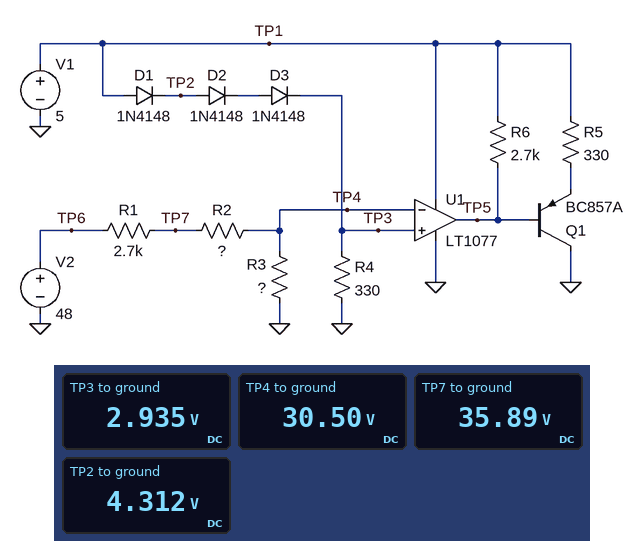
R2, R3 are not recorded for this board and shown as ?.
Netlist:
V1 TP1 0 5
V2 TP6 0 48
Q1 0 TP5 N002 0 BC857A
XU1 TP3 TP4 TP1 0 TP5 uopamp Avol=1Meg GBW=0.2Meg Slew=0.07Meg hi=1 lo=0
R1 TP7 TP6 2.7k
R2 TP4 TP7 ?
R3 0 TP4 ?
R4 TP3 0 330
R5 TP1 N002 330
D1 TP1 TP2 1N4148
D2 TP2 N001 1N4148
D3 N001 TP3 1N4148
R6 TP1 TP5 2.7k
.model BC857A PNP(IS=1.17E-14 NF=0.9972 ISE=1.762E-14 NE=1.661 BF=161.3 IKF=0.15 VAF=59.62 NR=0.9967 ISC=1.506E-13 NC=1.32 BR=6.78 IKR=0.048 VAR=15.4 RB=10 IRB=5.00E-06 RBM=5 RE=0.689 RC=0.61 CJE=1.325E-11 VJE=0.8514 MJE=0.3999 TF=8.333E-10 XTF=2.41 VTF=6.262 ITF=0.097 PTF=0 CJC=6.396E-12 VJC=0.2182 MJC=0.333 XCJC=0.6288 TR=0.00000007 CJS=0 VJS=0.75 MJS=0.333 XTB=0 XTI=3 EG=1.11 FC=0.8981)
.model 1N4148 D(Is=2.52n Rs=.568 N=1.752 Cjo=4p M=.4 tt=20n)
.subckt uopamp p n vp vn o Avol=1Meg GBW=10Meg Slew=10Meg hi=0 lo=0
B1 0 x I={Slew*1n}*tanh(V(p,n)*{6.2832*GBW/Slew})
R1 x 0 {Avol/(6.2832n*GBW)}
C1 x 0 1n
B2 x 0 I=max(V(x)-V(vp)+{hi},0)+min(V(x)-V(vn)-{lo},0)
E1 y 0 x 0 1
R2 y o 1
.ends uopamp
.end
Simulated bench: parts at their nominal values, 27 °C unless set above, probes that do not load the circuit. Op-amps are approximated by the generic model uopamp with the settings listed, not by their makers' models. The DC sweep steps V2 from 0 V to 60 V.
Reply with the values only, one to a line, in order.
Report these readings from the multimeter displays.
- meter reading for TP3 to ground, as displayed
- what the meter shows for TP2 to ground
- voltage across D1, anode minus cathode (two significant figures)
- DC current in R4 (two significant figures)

2.935 V
4.312 V
690 mV
8.9 mA
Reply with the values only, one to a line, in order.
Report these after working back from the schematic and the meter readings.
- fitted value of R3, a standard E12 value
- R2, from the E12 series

6.8 kΩ
1.2 kΩ
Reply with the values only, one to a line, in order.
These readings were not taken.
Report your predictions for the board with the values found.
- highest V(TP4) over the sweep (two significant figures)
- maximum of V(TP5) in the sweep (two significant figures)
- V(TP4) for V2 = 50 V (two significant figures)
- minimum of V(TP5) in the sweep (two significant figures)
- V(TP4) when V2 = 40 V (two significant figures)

38 V
4.0 V
32 V
1.9 mV
25 V
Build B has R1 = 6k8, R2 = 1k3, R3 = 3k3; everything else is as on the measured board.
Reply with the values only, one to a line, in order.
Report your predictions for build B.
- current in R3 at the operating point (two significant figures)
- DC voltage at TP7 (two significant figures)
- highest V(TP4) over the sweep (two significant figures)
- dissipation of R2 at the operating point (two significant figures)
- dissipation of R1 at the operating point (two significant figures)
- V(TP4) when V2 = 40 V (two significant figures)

4.2 mA
19 V
17 V
23 mW
120 mW
12 V
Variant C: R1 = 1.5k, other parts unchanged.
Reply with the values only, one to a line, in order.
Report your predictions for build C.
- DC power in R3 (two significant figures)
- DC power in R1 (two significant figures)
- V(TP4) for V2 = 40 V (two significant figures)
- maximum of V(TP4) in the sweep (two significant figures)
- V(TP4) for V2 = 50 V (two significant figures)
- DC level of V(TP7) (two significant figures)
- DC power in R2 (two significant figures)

170 mW
38 mW
29 V
43 V
36 V
40 V
31 mW
